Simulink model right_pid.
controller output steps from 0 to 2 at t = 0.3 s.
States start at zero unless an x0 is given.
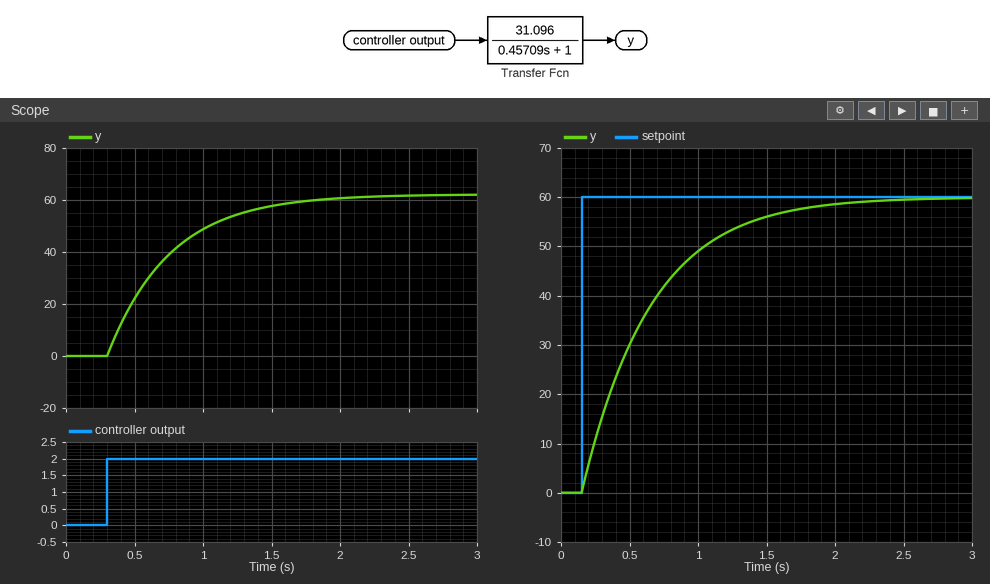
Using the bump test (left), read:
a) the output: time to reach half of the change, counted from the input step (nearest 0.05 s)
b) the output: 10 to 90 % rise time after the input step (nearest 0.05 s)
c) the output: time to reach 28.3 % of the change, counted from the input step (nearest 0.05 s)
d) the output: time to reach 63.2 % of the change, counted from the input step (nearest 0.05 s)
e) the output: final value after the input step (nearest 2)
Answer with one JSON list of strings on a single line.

["0.30 s", "1.00 s", "0.15 s", "0.45 s", "62"]
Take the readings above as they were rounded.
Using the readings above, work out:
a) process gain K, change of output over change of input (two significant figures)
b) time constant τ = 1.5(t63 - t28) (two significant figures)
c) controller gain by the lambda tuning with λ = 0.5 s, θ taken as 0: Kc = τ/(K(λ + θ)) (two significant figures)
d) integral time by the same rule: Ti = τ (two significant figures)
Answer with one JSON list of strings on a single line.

["31", "0.45 s", "0.029", "0.45 s"]
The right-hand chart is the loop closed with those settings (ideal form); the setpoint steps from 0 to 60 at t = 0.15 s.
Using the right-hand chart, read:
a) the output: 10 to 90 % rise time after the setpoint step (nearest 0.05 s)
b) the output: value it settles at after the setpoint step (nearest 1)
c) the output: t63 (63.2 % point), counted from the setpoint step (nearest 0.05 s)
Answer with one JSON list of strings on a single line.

["1.10 s", "60", "0.50 s"]
